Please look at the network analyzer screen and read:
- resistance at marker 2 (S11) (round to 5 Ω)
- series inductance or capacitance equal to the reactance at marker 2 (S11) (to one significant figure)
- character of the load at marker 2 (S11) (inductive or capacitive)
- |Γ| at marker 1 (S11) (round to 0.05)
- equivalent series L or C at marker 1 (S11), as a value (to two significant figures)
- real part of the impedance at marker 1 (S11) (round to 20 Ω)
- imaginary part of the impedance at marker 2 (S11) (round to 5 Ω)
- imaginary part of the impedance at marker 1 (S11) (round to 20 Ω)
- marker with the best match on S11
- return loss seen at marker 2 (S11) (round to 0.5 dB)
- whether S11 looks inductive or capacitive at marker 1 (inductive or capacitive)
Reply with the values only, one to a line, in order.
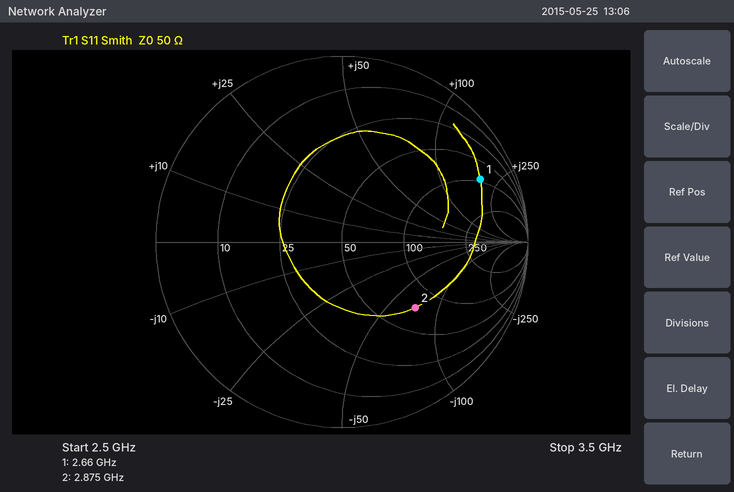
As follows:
75 Ω
800 fF
capacitive
0.80
11 nH
100 Ω
-70 Ω
+180 Ω
marker 2
5.5 dB
inductive
